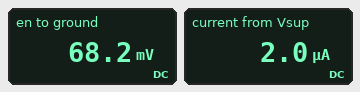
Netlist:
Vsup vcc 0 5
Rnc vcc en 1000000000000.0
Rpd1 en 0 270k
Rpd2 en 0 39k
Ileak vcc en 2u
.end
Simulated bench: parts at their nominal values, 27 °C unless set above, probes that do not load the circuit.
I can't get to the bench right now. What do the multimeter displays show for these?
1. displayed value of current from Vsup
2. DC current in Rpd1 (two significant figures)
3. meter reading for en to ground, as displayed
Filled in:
2.0 µA
250 nA
68.2 mV
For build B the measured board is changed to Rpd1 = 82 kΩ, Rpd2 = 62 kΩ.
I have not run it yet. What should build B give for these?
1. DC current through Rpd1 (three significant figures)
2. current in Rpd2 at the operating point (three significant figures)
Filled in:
861 nA
1.14 µA
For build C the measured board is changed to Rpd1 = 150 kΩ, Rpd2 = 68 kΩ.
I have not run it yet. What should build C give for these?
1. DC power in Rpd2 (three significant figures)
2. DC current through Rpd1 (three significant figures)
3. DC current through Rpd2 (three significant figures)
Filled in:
129 nW
624 nA
1.38 µA
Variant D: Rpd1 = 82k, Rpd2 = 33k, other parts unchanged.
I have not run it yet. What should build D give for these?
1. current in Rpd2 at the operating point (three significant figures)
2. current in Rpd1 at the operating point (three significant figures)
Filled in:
1.43 µA
574 nA
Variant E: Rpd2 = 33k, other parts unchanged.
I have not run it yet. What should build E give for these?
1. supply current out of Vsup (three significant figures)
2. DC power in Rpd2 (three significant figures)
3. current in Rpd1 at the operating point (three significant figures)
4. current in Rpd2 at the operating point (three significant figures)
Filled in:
2.00 µA
105 nW
218 nA
1.78 µA
